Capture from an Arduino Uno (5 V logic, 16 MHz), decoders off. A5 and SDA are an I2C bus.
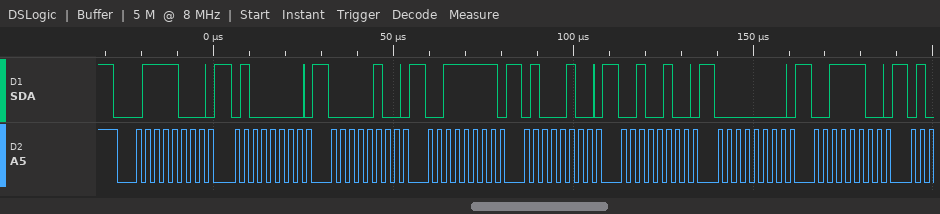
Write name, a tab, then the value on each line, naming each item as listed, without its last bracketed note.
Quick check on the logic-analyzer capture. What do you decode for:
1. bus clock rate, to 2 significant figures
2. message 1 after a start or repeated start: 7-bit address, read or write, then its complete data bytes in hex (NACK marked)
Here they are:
bus clock rate, to 2 significant figures	400 kHz
message 1 after a start or repeated start: 7-bit address, read or write, then its complete data bytes in hex	0x3C write: 40 04 3F 44 24 00 3C
